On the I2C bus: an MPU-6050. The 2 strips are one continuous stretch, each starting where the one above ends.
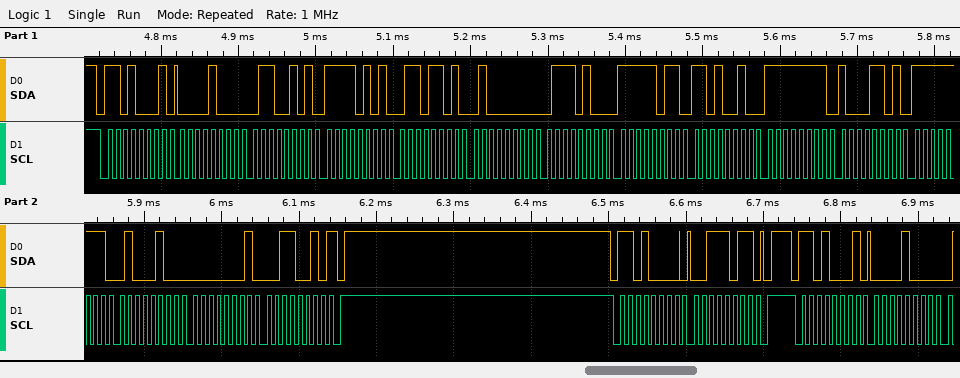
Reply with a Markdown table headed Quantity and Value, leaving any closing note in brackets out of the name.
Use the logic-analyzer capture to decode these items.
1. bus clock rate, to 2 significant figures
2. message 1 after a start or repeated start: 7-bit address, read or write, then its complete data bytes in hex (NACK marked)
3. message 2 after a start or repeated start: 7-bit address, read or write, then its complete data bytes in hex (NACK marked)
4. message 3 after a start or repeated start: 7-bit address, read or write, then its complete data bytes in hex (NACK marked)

| Quantity | Value |
|---|---|
| bus clock rate, to 2 significant figures | 100 kHz |
| message 1 after a start or repeated start: 7-bit address, read or write, then its complete data bytes in hex | 0x68 read: 08 65 F5 6D 40 74 FB D2 FF 8D FF 44 01 32 NACK |
| message 2 after a start or repeated start: 7-bit address, read or write, then its complete data bytes in hex | 0x68 write: 3B |
| message 3 after a start or repeated start: 7-bit address, read or write, then its complete data bytes in hex | 0x68 read: 08 |
